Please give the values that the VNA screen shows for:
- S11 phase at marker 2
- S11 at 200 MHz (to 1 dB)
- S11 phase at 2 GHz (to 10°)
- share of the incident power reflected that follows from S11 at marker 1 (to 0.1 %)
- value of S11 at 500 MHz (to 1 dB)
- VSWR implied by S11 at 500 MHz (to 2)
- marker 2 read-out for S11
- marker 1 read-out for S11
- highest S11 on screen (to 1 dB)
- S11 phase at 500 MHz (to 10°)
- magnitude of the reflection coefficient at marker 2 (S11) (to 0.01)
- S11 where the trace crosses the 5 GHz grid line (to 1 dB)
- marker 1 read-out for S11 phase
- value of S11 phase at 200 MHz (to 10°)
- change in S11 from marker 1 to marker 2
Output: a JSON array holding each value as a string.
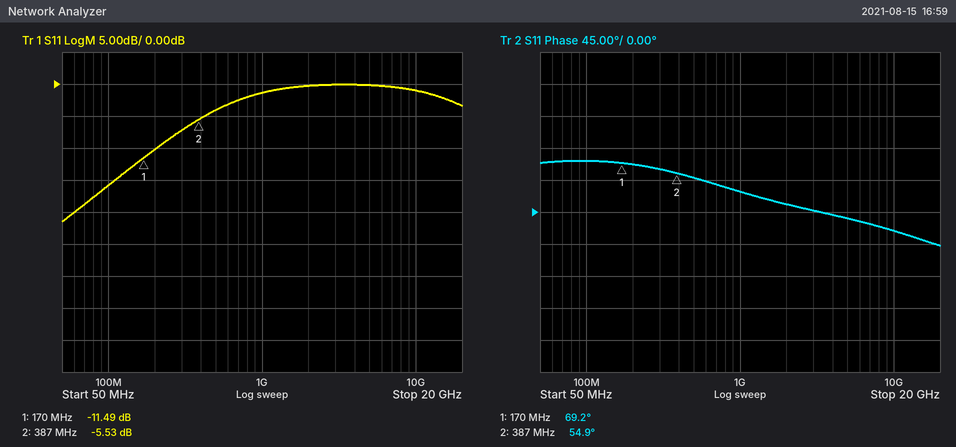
["54.9°", "-10 dB", "10°", "7.1 %", "-4 dB", "4", "-5.53 dB", "-11.49 dB", "0 dB", "50°", "0.53", "0 dB", "69.2°", "70°", "5.96 dB"]
